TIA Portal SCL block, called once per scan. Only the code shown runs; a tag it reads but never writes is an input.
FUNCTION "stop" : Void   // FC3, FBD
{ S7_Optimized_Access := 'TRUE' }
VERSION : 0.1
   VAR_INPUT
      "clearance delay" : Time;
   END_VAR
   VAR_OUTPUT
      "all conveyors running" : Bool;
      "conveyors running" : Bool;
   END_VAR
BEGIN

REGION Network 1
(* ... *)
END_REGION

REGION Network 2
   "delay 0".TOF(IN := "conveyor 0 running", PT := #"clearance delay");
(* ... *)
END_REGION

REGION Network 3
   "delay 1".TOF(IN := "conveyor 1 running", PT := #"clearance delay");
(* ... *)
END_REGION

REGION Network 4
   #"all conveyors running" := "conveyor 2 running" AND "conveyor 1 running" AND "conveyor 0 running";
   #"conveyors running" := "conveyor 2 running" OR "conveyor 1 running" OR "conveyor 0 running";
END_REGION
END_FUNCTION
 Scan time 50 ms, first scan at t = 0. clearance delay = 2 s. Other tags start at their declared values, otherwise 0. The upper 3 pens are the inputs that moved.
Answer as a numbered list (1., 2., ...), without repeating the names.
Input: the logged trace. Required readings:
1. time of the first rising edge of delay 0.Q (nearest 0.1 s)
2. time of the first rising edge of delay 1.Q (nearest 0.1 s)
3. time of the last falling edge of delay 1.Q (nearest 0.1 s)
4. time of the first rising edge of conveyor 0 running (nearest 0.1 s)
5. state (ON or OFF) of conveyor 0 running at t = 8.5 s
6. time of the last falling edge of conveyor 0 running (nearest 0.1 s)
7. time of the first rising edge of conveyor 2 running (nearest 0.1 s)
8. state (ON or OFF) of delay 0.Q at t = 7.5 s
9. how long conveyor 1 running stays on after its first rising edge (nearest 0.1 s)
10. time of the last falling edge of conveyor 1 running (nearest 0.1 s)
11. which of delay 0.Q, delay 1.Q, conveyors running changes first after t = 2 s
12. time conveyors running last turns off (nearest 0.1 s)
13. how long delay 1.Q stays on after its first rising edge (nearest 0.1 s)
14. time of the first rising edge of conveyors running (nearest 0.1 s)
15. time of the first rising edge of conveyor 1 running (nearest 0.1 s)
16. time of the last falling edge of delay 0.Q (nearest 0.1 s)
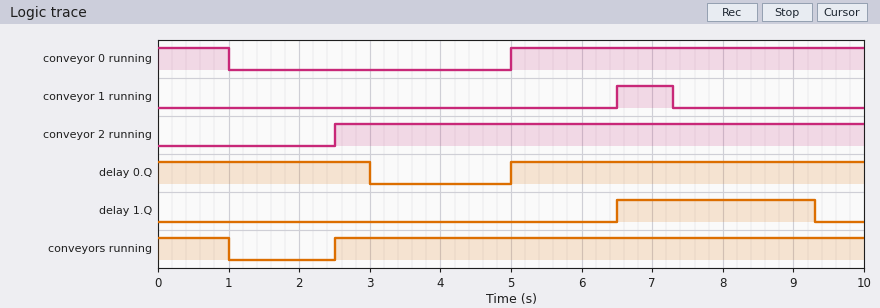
1. 5.0 s
2. 6.5 s
3. 9.3 s
4. 5.0 s
5. ON
6. 1.0 s
7. 2.5 s
8. ON
9. 0.8 s
10. 7.3 s
11. conveyors running
12. 1.0 s
13. 2.8 s
14. 2.5 s
15. 6.5 s
16. 3.0 s
